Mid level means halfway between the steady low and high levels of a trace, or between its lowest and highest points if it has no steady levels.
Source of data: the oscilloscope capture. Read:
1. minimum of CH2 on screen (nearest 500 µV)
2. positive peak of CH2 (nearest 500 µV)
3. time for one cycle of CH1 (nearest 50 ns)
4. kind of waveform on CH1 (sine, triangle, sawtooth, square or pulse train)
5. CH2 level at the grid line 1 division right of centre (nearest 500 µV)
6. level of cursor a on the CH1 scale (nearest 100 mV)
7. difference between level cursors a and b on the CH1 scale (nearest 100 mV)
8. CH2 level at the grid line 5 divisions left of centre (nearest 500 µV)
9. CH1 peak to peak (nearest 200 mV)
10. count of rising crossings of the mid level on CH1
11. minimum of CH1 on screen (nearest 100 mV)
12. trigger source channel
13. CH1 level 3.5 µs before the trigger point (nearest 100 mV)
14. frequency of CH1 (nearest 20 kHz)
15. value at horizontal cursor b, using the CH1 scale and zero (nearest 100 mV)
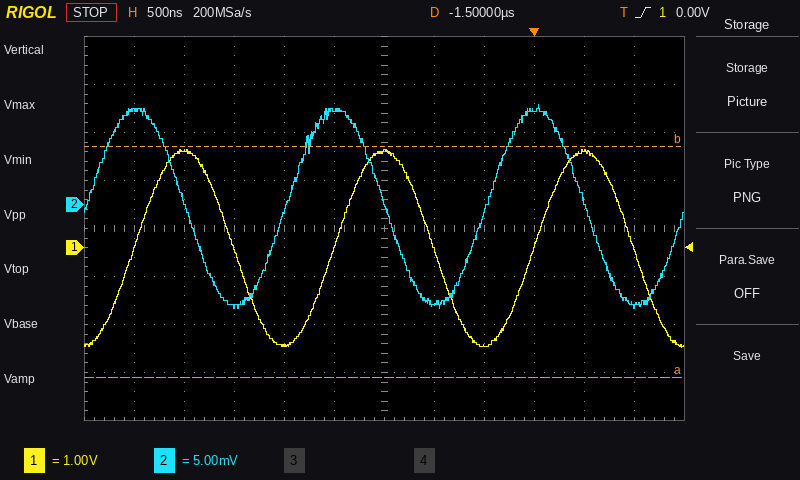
-11.0 mV
10.5 mV
2.00 µs
sine
-10.5 mV
-2.7 V
4.8 V
10.0 mV
4.2 V
3
-2.1 V
CH1
2.0 V
500 kHz
2.1 V
